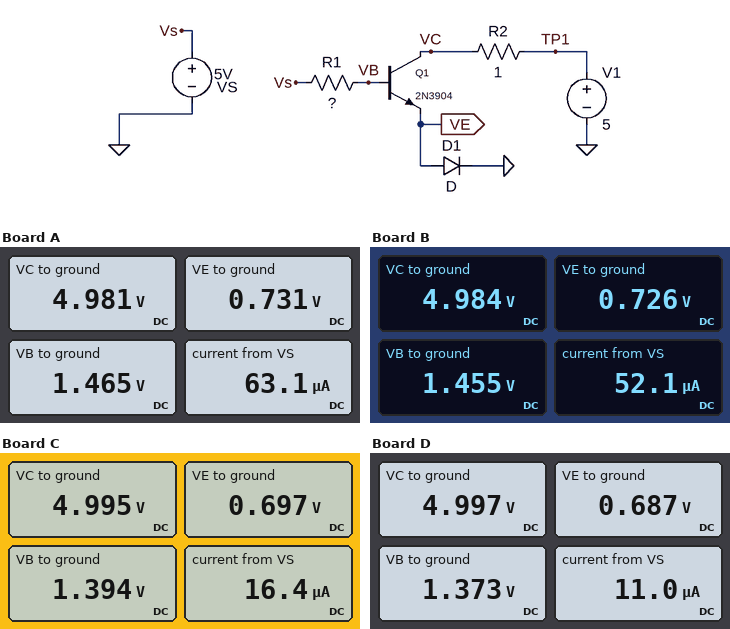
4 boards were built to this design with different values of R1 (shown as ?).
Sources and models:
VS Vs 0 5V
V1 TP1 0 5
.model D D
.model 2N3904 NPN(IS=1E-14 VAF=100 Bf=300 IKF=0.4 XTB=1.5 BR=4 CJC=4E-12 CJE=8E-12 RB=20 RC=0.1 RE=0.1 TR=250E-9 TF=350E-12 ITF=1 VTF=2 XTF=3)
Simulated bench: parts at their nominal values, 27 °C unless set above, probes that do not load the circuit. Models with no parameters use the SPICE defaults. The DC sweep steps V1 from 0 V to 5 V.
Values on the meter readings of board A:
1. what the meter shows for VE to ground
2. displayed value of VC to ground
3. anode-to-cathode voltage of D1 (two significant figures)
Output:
0.731 V
4.981 V
730 mV
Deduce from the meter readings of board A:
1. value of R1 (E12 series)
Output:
56 kΩ
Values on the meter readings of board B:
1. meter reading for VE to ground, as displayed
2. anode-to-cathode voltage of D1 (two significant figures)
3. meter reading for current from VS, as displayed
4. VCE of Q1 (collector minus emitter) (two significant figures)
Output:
0.726 V
730 mV
52.1 µA
4.3 V
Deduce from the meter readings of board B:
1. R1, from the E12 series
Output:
68 kΩ
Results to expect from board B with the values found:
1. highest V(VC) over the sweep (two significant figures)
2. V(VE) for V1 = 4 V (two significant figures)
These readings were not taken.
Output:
5.0 V
730 mV
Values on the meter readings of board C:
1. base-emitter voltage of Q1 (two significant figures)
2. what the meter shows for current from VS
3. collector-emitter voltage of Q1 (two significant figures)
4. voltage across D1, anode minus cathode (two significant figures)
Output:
700 mV
16.4 µA
4.3 V
700 mV
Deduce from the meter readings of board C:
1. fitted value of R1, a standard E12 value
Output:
220 kΩ
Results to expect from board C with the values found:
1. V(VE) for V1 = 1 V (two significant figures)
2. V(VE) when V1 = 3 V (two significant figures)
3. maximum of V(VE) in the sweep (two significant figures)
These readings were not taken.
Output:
700 mV
700 mV
700 mV
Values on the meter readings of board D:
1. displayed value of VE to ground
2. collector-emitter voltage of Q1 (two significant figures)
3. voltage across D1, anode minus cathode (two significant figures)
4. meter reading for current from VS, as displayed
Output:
0.687 V
4.3 V
690 mV
11.0 µA
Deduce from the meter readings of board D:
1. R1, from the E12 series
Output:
330 kΩ
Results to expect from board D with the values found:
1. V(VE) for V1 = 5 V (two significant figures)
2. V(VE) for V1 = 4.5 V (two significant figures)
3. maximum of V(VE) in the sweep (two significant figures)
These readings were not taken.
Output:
690 mV
690 mV
690 mV
